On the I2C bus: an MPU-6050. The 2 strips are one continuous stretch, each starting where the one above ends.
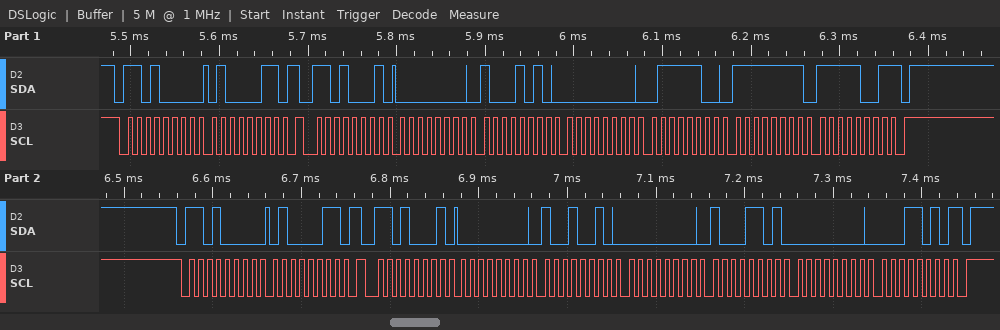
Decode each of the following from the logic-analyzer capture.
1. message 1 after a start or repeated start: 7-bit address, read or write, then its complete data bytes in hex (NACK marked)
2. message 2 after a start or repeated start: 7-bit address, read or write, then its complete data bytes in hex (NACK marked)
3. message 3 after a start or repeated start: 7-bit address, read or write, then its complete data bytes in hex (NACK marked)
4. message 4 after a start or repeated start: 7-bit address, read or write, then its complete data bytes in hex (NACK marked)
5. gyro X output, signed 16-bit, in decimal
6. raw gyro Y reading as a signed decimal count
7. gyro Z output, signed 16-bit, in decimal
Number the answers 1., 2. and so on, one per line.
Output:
1. 0x68 write: 43
2. 0x68 read: 00 8A 00 7C FF F9 NACK
3. 0x68 write: 43
4. 0x68 read: 00 92 00 8D 00 1A NACK
5. 138
6. 124
7. -7
